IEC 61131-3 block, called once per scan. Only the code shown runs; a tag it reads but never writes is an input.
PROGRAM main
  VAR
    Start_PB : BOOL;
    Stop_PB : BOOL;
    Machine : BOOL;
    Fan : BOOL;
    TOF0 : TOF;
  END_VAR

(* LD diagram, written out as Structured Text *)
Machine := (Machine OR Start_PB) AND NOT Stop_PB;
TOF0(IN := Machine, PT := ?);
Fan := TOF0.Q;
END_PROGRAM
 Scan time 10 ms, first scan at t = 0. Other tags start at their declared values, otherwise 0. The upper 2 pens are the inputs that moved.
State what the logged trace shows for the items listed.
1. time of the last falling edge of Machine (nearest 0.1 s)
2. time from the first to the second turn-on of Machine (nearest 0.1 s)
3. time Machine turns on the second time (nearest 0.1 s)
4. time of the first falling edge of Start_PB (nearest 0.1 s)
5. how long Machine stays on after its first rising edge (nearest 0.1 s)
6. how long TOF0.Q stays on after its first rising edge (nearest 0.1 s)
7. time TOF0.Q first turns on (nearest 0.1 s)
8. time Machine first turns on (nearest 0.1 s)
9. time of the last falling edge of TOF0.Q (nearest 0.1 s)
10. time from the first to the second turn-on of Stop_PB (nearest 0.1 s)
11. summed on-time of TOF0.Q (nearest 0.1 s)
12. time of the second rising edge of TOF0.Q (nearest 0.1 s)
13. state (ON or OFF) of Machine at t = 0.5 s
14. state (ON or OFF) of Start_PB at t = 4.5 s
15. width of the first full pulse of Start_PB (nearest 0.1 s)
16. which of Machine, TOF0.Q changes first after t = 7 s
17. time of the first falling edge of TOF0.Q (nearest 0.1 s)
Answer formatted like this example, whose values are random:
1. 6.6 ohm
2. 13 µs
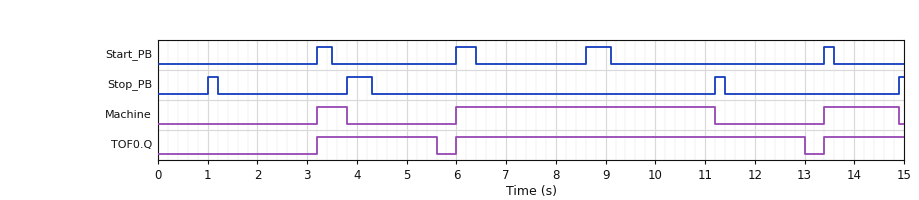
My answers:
1. 14.9 s
2. 2.8 s
3. 6.0 s
4. 3.5 s
5. 0.6 s
6. 2.4 s
7. 3.2 s
8. 3.2 s
9. 13.0 s
10. 2.8 s
11. 11.0 s
12. 6.0 s
13. OFF
14. OFF
15. 0.3 s
16. Machine
17. 5.6 s
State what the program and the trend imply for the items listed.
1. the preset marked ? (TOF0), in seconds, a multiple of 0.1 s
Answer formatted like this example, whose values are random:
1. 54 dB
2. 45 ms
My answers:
1. 1.8 s
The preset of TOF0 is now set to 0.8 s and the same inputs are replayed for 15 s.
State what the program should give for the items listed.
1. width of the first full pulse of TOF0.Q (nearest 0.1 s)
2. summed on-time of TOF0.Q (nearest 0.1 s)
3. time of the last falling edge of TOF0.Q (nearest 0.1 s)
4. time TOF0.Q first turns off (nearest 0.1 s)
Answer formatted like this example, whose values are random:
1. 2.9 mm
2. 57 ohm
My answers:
1. 1.4 s
2. 9.0 s
3. 12.0 s
4. 4.6 s
